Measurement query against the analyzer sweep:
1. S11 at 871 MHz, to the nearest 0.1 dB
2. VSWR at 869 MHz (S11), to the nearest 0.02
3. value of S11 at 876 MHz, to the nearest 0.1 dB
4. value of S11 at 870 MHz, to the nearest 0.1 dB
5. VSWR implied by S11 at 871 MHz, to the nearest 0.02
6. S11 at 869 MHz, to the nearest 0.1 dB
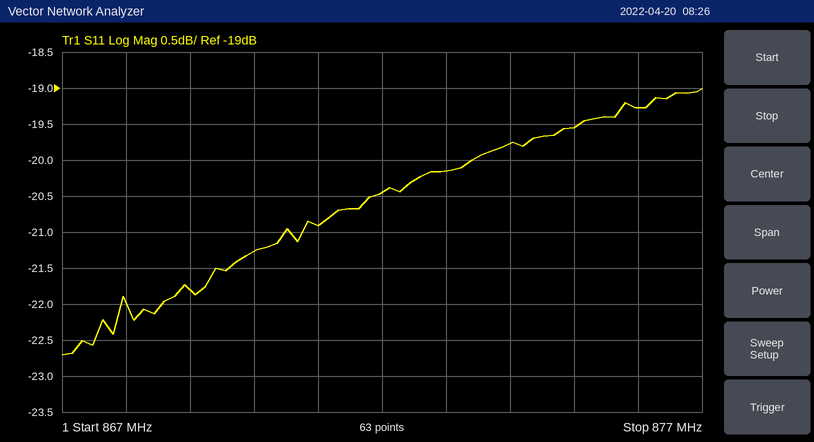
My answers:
-20.9 dB
1.18
-19.3 dB
-21.3 dB
1.20
-21.8 dB
